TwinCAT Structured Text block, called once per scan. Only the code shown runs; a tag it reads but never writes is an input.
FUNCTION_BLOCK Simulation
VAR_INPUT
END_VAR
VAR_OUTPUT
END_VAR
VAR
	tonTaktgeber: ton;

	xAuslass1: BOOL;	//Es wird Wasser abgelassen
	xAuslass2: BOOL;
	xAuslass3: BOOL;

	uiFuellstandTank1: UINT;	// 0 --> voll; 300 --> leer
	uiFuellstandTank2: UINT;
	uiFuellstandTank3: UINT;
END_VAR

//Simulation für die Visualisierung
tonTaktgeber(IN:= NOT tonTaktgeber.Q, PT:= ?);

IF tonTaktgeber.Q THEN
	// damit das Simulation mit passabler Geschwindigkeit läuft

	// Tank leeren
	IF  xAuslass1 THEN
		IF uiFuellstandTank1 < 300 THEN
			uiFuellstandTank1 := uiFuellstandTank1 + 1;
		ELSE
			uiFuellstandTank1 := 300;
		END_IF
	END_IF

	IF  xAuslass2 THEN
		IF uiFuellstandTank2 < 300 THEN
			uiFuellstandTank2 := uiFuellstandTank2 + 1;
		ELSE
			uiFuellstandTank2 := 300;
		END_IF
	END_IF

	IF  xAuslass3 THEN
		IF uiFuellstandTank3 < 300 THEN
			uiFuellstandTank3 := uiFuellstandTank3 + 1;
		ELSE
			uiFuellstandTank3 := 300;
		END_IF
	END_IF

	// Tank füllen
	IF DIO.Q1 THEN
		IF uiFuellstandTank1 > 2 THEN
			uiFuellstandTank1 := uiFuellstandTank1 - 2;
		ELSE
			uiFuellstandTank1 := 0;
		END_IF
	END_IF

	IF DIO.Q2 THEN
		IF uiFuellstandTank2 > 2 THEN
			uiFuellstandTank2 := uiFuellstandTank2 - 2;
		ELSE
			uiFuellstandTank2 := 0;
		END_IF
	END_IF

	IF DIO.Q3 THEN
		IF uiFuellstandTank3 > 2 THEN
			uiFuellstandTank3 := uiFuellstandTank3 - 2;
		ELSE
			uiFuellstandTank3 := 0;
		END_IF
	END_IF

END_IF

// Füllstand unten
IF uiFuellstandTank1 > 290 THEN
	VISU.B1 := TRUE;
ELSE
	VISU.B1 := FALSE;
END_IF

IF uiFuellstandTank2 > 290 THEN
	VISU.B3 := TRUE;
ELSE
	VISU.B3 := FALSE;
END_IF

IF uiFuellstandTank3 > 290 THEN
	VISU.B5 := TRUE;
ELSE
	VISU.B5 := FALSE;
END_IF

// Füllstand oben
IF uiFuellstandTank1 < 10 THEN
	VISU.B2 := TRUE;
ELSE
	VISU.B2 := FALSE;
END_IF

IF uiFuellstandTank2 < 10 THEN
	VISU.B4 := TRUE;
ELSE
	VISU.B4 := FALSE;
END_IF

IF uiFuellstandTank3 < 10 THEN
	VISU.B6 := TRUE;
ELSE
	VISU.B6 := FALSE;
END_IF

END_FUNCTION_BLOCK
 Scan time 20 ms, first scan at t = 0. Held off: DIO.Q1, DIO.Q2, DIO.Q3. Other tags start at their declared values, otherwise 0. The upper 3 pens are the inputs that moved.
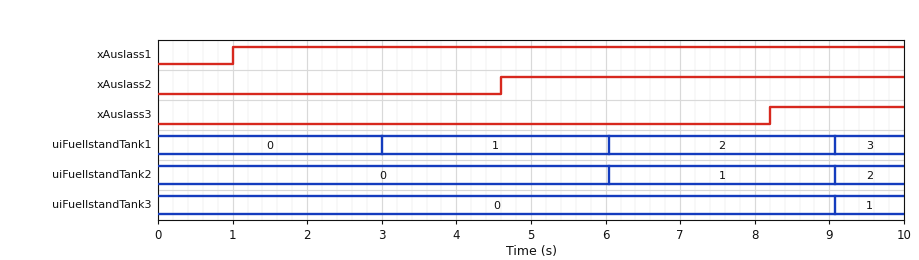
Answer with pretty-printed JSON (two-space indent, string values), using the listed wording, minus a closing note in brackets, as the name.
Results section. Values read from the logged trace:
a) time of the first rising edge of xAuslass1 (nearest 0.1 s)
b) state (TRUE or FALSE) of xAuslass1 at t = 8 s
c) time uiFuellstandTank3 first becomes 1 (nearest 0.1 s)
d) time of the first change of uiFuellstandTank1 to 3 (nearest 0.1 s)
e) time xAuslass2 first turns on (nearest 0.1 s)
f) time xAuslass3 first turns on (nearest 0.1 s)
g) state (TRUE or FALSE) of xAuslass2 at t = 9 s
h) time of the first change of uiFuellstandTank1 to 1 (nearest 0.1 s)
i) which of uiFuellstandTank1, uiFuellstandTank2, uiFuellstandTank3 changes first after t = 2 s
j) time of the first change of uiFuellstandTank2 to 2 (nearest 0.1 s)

{
  "time of the first rising edge of xAuslass1": "1.0 s",
  "state (TRUE or FALSE) of xAuslass1 at t = 8 s": "TRUE",
  "time uiFuellstandTank3 first becomes 1": "9.1 s",
  "time of the first change of uiFuellstandTank1 to 3": "9.1 s",
  "time xAuslass2 first turns on": "4.6 s",
  "time xAuslass3 first turns on": "8.2 s",
  "state (TRUE or FALSE) of xAuslass2 at t = 9 s": "TRUE",
  "time of the first change of uiFuellstandTank1 to 1": "3.0 s",
  "which of uiFuellstandTank1, uiFuellstandTank2, uiFuellstandTank3 changes first after t = 2 s": "uiFuellstandTank1",
  "time of the first change of uiFuellstandTank2 to 2": "9.1 s"
}
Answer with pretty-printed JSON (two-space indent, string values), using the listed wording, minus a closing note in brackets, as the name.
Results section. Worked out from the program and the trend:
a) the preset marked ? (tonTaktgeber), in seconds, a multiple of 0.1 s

{
  "the preset marked ? (tonTaktgeber), in seconds, a multiple of 0.1 s": "3.0 s"
}
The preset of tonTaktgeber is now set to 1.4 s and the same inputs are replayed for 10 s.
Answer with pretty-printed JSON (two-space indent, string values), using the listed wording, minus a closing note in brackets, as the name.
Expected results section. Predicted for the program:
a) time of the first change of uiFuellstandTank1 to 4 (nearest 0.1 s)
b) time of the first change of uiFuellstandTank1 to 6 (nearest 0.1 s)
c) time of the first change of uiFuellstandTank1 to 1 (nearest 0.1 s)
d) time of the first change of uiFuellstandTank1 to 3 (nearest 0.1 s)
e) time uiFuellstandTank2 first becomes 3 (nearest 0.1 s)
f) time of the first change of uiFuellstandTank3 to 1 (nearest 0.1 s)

{
  "time of the first change of uiFuellstandTank1 to 4": "5.7 s",
  "time of the first change of uiFuellstandTank1 to 6": "8.6 s",
  "time of the first change of uiFuellstandTank1 to 1": "1.4 s",
  "time of the first change of uiFuellstandTank1 to 3": "4.3 s",
  "time uiFuellstandTank2 first becomes 3": "8.6 s",
  "time of the first change of uiFuellstandTank3 to 1": "8.6 s"
}
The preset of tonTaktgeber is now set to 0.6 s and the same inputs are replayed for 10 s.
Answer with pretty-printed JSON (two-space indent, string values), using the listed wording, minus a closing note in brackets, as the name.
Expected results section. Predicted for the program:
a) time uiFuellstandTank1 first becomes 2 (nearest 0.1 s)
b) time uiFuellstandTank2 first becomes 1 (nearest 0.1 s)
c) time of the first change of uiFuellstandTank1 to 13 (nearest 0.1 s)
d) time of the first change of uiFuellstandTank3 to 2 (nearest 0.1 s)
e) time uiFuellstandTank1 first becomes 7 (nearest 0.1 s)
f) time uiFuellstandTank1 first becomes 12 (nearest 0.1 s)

{
  "time uiFuellstandTank1 first becomes 2": "1.9 s",
  "time uiFuellstandTank2 first becomes 1": "5.1 s",
  "time of the first change of uiFuellstandTank1 to 13": "8.9 s",
  "time of the first change of uiFuellstandTank3 to 2": "8.9 s",
  "time uiFuellstandTank1 first becomes 7": "5.1 s",
  "time uiFuellstandTank1 first becomes 12": "8.3 s"
}
